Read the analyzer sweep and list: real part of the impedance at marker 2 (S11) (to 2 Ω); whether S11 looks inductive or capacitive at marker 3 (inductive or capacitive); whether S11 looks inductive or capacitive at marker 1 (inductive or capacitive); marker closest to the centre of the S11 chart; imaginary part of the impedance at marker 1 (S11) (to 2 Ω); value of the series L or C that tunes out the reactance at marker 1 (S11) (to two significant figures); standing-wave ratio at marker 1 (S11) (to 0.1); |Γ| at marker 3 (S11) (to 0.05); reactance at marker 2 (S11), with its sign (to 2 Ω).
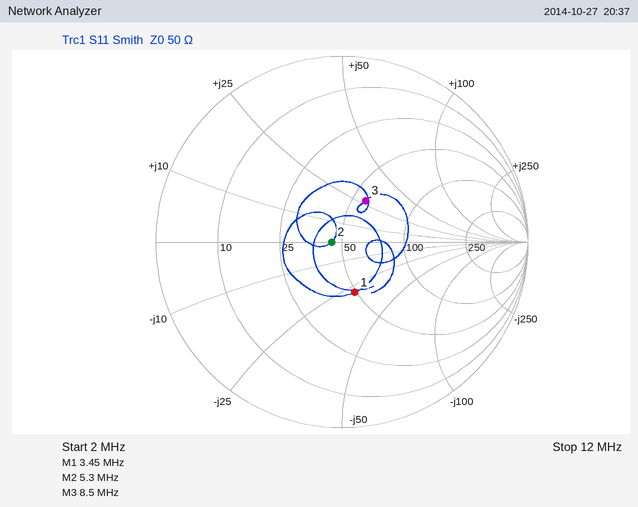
44 Ω
inductive
capacitive
marker 2
-28 Ω
1.3 µH
1.8
0.25
0 Ω
